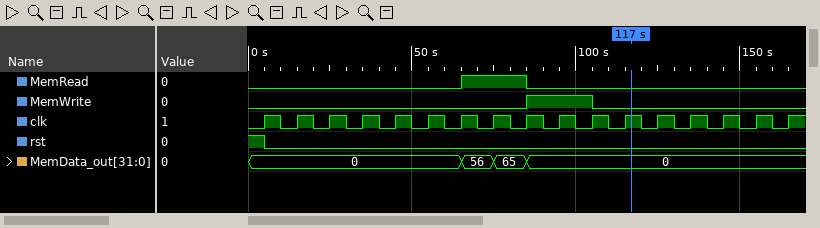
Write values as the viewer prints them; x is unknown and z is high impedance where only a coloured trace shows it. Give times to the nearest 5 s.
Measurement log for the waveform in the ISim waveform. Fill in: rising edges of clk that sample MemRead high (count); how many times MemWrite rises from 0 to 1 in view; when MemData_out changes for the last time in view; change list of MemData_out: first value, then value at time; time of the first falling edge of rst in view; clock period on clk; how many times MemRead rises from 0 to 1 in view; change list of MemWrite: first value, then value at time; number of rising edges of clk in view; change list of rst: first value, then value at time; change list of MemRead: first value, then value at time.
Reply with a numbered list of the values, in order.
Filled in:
1. 2
2. 1
3. 85 s
4. 0, 56 at 65 s, 65 at 75 s, 0 at 85 s
5. 5 s
6. 10 s
7. 1
8. 0, 1 at 85 s, 0 at 105 s
9. 17
10. 1, 0 at 5 s
11. 0, 1 at 65 s, 0 at 85 s
